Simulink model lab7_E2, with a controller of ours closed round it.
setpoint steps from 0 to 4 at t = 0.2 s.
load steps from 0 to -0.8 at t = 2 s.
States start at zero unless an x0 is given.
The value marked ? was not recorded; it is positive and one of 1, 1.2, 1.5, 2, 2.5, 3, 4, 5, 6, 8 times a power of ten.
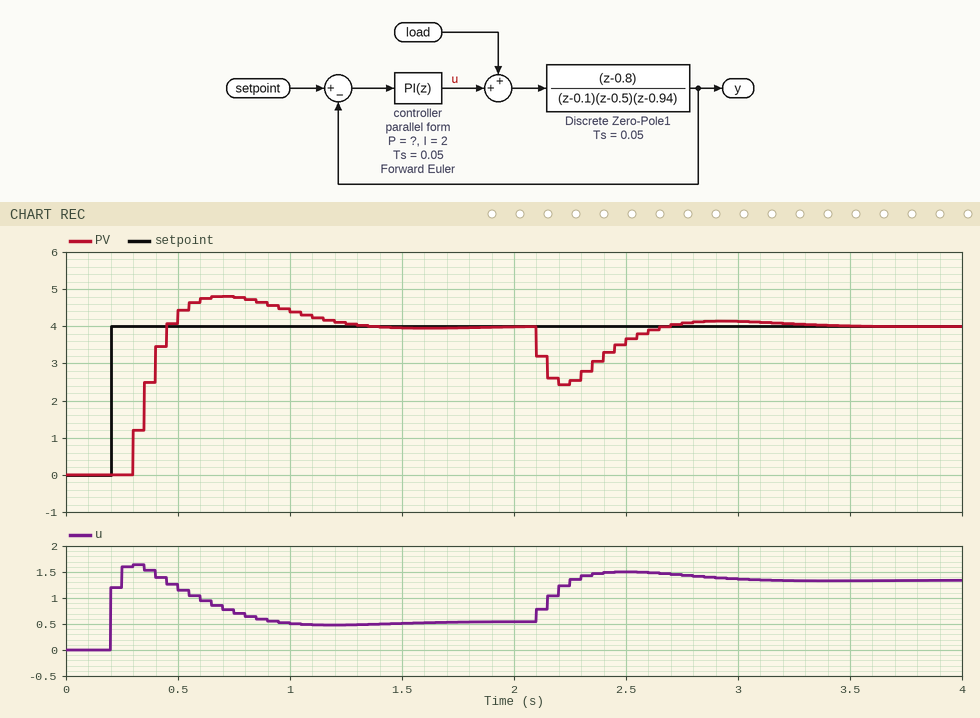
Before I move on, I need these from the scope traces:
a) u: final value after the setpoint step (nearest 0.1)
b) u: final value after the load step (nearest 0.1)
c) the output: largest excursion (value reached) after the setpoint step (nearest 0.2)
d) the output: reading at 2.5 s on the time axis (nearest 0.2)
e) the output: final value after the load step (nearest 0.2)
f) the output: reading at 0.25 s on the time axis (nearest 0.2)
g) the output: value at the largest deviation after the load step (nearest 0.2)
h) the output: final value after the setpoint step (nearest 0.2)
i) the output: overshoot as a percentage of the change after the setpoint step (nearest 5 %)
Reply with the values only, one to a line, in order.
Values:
0.5
1.3
4.8
3.6
4.0
0.0
2.4
4.0
20 %
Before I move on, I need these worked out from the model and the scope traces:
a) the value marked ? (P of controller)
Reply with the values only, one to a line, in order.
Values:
0.3
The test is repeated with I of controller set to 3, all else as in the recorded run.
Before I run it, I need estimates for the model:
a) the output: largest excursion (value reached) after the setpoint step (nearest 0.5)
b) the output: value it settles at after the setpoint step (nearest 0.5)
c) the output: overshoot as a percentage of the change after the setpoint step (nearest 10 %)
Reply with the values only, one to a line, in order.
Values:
5.5
4.0
40 %
